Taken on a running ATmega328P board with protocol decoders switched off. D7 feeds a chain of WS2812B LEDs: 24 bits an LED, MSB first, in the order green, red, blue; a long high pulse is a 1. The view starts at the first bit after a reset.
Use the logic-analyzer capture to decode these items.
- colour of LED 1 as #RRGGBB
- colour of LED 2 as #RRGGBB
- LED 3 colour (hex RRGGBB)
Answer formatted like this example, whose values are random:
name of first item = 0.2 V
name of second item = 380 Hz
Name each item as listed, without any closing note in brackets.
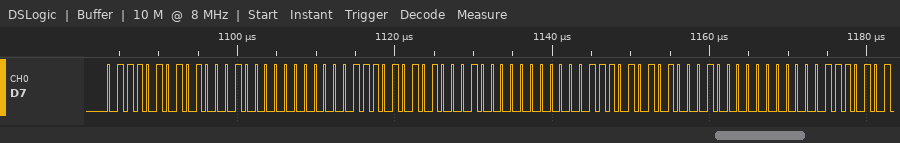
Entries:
colour of LED 1 as #RRGGBB = #447500
colour of LED 2 as #RRGGBB = #447500
LED 3 colour = #447500
